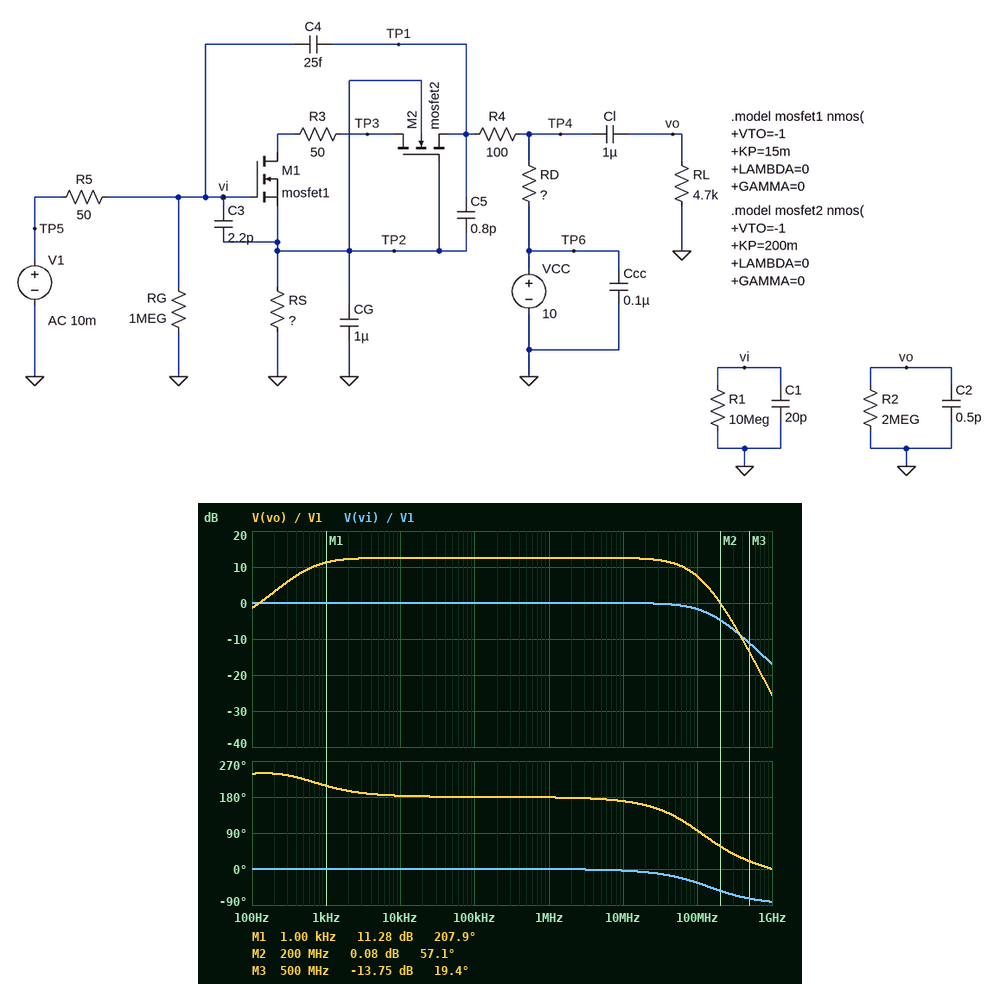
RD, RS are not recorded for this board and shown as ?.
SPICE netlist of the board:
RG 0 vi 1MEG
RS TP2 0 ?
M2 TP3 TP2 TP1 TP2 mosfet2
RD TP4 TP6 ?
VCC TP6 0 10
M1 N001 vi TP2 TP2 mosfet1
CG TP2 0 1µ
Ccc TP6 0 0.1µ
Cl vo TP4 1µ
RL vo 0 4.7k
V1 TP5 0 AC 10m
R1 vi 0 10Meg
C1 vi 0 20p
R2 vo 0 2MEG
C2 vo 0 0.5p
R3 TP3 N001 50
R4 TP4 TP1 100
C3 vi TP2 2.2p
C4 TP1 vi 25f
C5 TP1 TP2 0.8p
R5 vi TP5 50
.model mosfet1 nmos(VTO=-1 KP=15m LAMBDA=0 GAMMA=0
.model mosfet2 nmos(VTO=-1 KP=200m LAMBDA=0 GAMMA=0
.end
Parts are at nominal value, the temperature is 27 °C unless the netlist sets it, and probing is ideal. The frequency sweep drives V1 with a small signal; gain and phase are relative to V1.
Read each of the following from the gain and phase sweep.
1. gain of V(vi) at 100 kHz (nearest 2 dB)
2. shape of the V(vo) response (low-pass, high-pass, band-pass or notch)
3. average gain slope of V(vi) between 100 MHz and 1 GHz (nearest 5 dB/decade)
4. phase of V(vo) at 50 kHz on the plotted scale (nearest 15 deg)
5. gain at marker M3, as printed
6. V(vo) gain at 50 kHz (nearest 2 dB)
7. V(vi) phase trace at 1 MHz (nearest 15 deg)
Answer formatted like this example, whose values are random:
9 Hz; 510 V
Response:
0 dB; band-pass; -15 dB/decade; 180 deg; -13.75 dB; 12 dB; 0 deg
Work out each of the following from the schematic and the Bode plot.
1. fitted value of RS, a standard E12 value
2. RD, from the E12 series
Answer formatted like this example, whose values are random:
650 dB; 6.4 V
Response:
2.2 kΩ; 1.8 kΩ
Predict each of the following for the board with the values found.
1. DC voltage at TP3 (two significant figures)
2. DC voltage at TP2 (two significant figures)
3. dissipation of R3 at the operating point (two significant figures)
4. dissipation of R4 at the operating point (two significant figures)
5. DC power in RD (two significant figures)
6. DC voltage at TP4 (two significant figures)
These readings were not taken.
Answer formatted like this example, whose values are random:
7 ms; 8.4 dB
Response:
1.7 V; 780 mV; 6.3 µW; 13 µW; 230 µW; 9.4 V
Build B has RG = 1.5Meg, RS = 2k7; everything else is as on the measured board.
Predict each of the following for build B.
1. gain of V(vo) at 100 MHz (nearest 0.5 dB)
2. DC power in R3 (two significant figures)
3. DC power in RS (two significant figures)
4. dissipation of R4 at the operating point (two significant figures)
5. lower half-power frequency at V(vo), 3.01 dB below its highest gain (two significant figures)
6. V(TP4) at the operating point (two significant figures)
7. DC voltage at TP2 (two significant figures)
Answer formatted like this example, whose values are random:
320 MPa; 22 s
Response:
6.5 dB; 4.4 µW; 240 µW; 8.8 µW; 530 Hz; 9.5 V; 800 mV
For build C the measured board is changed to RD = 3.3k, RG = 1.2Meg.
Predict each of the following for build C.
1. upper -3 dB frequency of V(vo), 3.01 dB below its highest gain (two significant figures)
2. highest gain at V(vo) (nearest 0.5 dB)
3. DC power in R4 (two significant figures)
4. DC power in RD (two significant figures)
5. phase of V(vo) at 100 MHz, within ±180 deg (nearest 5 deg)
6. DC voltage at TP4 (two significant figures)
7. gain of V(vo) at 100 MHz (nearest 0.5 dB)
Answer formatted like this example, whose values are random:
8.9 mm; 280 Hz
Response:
53 MHz; 16.0 dB; 13 µW; 420 µW; 85 deg; 8.8 V; 8.5 dB
